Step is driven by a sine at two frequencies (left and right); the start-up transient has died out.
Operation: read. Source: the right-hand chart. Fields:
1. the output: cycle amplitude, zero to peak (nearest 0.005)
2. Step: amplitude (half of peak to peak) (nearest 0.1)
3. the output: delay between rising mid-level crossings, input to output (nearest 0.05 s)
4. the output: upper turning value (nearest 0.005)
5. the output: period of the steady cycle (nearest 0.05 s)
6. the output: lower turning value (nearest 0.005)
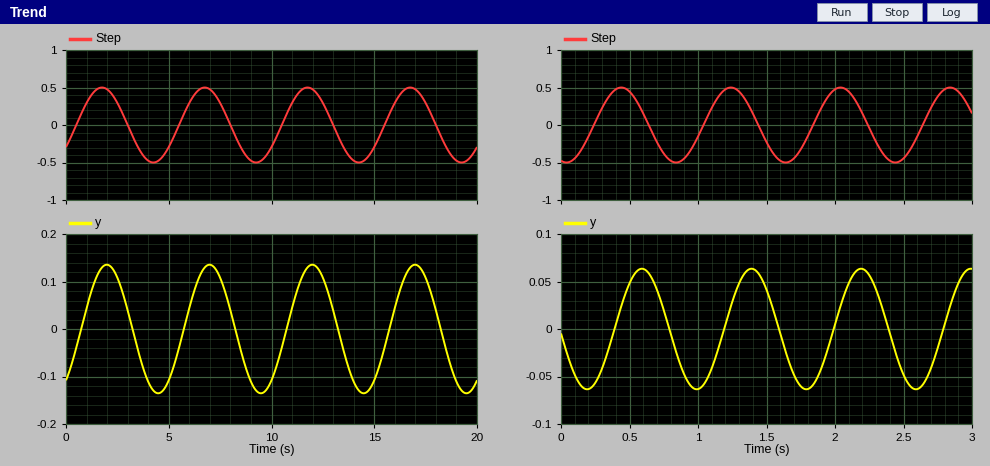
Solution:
0.065
0.5
0.15 s
0.065
0.80 s
-0.065
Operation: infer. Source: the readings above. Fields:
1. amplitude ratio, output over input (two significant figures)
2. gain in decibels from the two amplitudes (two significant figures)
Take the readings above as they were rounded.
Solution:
0.13
-18 dB
